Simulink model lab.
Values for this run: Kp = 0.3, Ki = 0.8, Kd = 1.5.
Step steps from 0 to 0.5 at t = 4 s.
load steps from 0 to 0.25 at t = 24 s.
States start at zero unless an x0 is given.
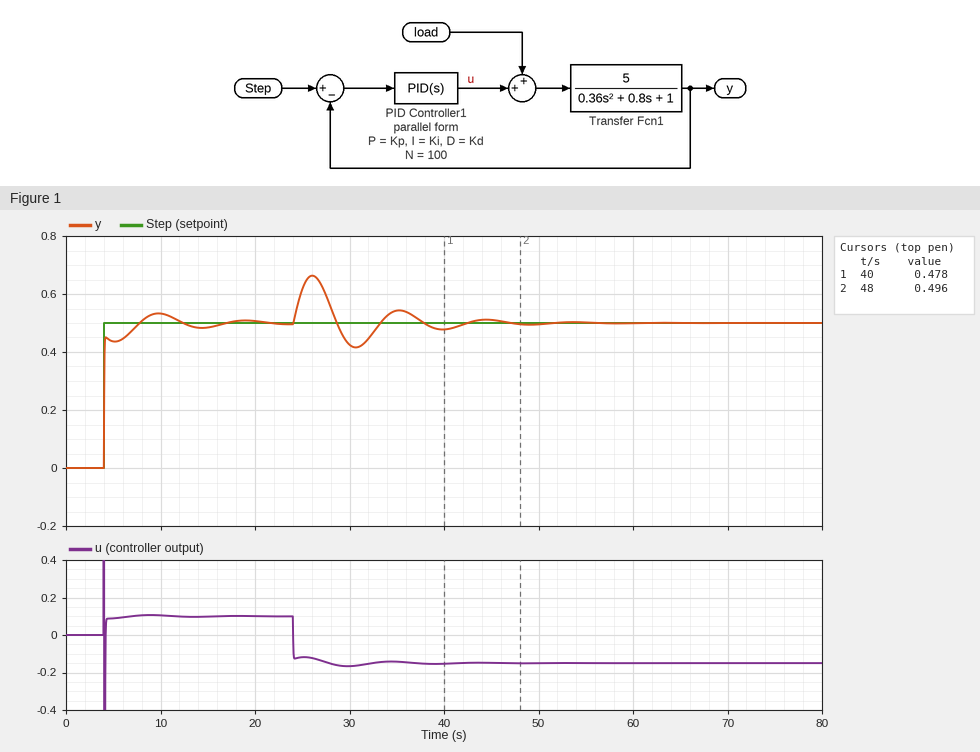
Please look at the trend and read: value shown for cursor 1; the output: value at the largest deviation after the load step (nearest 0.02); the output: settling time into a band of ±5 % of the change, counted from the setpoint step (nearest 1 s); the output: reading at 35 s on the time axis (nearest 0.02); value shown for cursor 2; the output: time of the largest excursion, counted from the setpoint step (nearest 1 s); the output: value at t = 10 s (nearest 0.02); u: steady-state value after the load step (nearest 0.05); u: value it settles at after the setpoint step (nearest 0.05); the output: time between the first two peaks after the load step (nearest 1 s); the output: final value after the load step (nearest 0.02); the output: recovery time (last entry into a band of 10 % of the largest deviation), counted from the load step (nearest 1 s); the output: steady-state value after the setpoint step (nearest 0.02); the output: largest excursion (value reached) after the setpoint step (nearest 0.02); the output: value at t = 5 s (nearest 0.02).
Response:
0.478
0.66
7 s
0.54
0.496
6 s
0.54
-0.15
0.10
9 s
0.50
17 s
0.50
0.54
0.44
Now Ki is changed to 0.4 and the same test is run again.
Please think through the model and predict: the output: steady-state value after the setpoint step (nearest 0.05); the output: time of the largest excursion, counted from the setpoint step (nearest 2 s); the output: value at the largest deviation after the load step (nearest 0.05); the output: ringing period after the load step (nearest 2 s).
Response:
0.50
8 s
0.70
14 s
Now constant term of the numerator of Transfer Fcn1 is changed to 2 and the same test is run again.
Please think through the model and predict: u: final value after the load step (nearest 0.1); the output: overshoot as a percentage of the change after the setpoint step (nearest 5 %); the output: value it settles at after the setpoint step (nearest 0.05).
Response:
0.0
10 %
0.50
